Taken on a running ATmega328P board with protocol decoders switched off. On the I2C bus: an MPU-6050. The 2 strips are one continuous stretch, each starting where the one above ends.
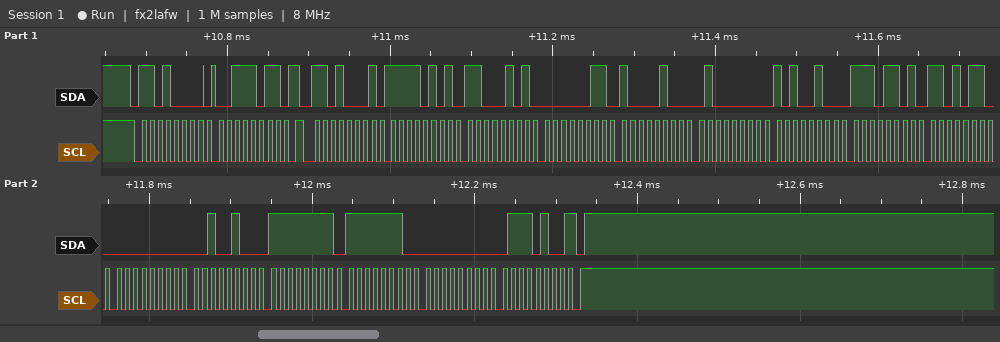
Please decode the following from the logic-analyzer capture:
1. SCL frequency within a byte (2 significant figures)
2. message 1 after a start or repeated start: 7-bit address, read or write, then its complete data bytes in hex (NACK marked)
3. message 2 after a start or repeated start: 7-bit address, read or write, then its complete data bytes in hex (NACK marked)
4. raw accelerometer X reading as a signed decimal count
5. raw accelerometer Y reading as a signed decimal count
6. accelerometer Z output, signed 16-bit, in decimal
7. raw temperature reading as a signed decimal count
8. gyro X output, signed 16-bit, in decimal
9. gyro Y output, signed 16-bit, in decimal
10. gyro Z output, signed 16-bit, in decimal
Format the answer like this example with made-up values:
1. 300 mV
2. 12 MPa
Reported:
1. 100 kHz
2. 0x68 write: 3B
3. 0x68 read: F5 C5 03 84 40 A4 ED D6 00 24 FF FE 00 74 NACK
4. -2619
5. 900
6. 16548
7. -4650
8. 36
9. -2
10. 116
